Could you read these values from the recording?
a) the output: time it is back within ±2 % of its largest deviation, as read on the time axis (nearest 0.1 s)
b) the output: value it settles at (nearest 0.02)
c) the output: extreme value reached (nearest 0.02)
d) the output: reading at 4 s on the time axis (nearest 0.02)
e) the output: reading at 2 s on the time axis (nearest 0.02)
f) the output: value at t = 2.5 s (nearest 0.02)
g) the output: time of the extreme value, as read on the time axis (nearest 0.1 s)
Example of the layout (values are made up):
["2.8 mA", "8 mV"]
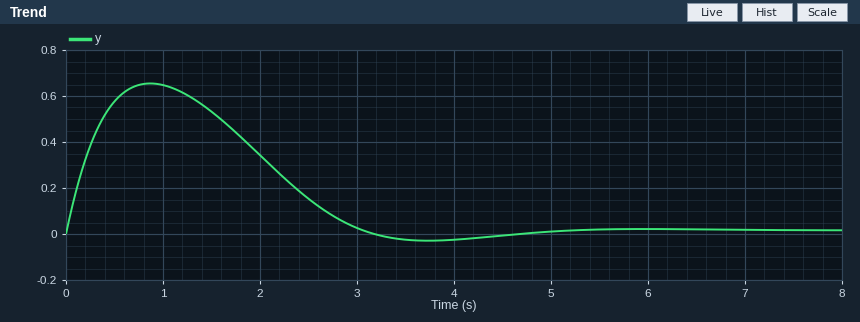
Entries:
["4.8 s", "0.02", "0.66", "-0.02", "0.34", "0.16", "0.9 s"]
